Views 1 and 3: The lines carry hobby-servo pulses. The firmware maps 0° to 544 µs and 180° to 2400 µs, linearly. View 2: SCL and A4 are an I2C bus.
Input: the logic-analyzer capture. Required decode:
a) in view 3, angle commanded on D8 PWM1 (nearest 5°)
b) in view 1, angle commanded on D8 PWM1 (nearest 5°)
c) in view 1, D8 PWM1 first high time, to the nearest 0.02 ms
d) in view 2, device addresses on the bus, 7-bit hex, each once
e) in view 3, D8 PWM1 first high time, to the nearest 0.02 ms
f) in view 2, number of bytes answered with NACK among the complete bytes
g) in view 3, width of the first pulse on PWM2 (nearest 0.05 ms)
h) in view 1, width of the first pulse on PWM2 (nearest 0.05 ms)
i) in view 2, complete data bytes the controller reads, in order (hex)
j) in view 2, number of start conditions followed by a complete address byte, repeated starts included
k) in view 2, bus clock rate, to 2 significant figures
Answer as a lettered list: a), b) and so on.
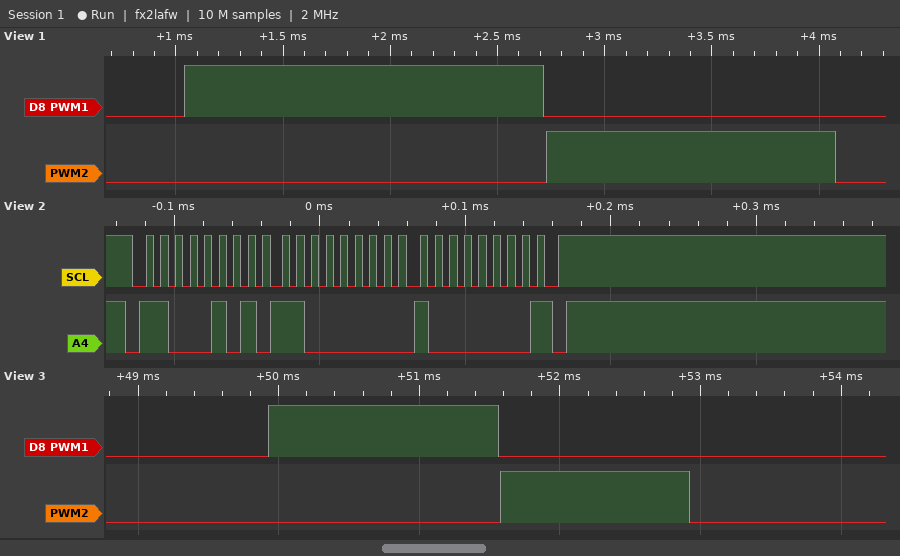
a) 105°
b) 110°
c) 1.68 ms
d) 0x62
e) 1.64 ms
f) 1
g) 1.35 ms
h) 1.35 ms
i) C0 80
j) 1
k) 100 kHz
